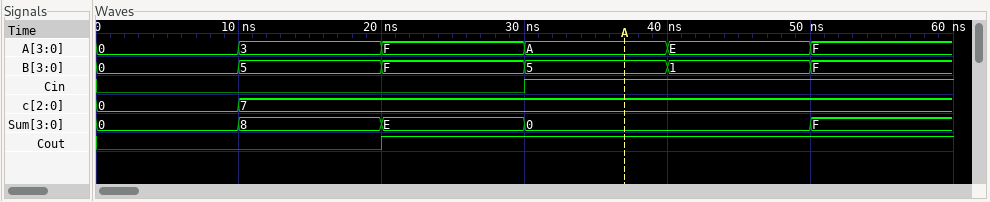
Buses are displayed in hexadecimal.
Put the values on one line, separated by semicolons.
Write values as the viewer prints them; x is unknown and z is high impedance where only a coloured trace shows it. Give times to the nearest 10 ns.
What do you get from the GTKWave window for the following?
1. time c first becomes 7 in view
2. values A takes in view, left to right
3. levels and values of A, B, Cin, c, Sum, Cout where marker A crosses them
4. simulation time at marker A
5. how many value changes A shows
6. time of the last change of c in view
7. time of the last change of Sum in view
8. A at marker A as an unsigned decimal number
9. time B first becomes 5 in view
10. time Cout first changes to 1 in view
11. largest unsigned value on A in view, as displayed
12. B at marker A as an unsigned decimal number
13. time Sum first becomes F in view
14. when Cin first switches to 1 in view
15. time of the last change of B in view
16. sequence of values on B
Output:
10 ns; 0, 3, F, A, E, F; A=A, B=5, Cin=1, c=7, Sum=0, Cout=1; 40 ns; 5; 10 ns; 50 ns; 10; 10 ns; 20 ns; F; 5; 50 ns; 30 ns; 50 ns; 0, 5, F, 5, 1, F
